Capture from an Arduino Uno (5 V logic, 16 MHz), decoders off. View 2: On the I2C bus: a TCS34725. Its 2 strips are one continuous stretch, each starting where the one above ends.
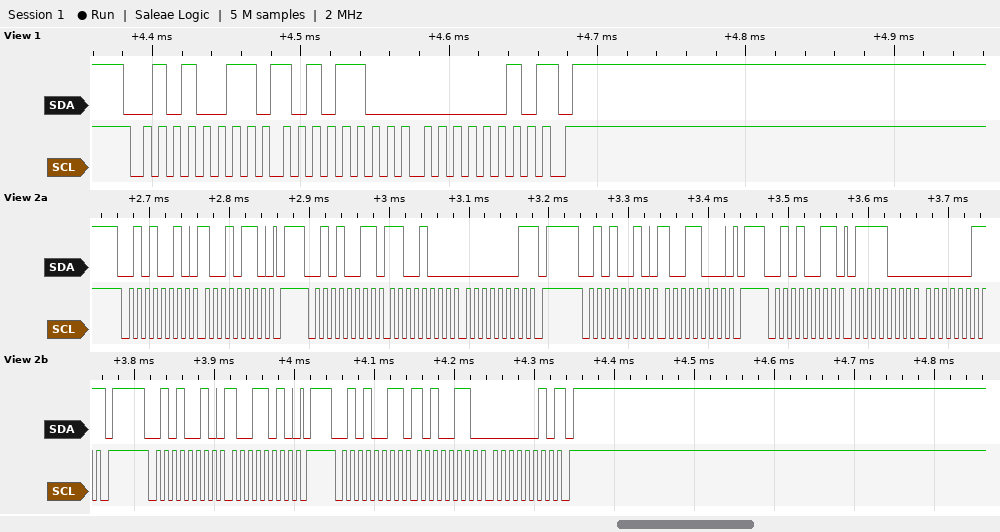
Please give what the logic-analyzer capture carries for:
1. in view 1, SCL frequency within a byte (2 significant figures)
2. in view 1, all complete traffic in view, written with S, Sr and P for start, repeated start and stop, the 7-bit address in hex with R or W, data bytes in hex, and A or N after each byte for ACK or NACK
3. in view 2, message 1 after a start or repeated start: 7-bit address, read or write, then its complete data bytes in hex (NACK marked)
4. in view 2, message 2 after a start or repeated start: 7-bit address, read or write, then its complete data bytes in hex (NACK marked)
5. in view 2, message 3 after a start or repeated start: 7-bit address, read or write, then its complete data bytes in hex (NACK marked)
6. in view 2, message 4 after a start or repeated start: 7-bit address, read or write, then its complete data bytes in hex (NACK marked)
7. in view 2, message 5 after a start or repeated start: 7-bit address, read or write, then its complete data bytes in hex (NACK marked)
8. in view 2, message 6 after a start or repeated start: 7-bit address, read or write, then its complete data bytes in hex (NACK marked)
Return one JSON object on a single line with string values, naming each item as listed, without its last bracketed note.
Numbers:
{"in view 1, SCL frequency within a byte": "100 kHz", "in view 1, all complete traffic in view, written with S, Sr and P for start, repeated start and stop, the 7-bit address in hex with R or W, data bytes in hex, and A or N after each byte for ACK or NACK": "S 29R A AC A 02 N P", "in view 2, message 1 after a start or repeated start: 7-bit address, read or write, then its complete data bytes in hex": "0x29 write: 96", "in view 2, message 2 after a start or repeated start: 7-bit address, read or write, then its complete data bytes in hex": "0x29 read: C8 01 NACK", "in view 2, message 3 after a start or repeated start: 7-bit address, read or write, then its complete data bytes in hex": "0x29 write: 98", "in view 2, message 4 after a start or repeated start: 7-bit address, read or write, then its complete data bytes in hex": "0x29 read: 78 03 NACK", "in view 2, message 5 after a start or repeated start: 7-bit address, read or write, then its complete data bytes in hex": "0x29 write: 9A", "in view 2, message 6 after a start or repeated start: 7-bit address, read or write, then its complete data bytes in hex": "0x29 read: A6 02 NACK"}
